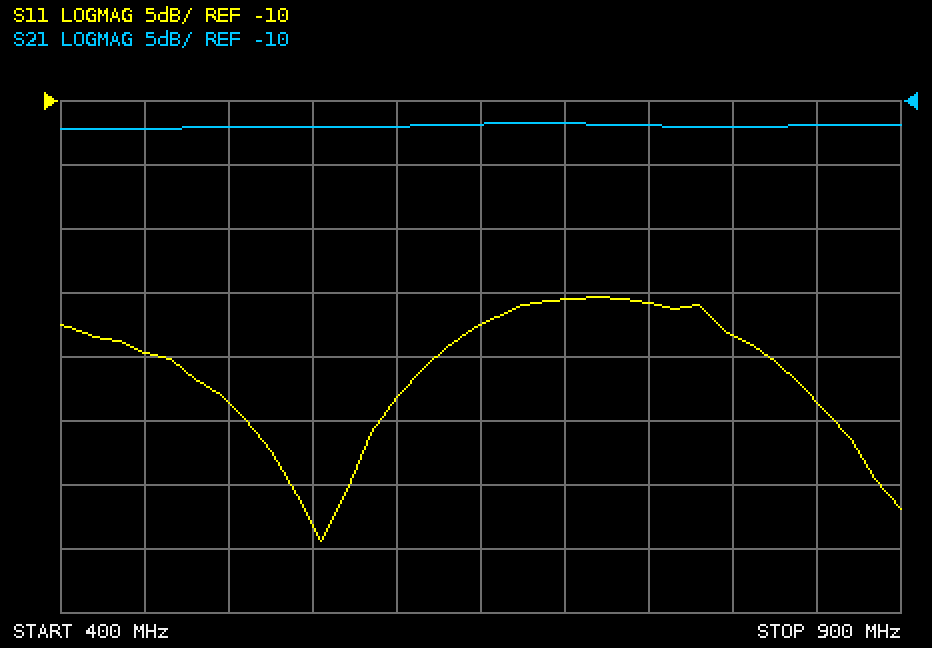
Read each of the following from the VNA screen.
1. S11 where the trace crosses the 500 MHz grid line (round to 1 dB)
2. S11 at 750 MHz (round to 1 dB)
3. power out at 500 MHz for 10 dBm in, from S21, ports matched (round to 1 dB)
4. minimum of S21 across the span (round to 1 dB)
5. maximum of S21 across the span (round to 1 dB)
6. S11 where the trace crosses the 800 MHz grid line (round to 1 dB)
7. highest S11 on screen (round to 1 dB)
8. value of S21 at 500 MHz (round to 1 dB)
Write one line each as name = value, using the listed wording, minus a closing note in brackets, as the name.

S11 where the trace crosses the 500 MHz grid line = -34 dB
S11 at 750 MHz = -26 dB
power out at 500 MHz for 10 dBm in, from S21, ports matched = -2 dBm
minimum of S21 across the span = -12 dB
maximum of S21 across the span = -12 dB
S11 where the trace crosses the 800 MHz grid line = -28 dB
highest S11 on screen = -25 dB
value of S21 at 500 MHz = -12 dB
